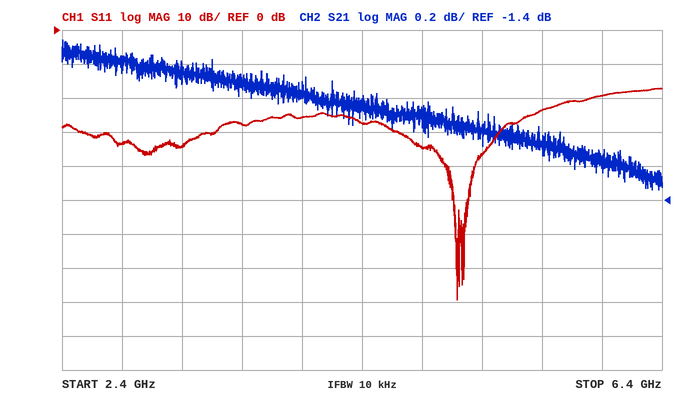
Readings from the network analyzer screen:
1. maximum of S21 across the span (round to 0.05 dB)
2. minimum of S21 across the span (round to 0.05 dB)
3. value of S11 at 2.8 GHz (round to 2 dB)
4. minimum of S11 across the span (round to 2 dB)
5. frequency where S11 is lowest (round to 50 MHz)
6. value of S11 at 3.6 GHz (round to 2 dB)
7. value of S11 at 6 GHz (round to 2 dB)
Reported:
-0.45 dB
-1.35 dB
-34 dB
-80 dB
5.05 GHz
-28 dB
-20 dB
